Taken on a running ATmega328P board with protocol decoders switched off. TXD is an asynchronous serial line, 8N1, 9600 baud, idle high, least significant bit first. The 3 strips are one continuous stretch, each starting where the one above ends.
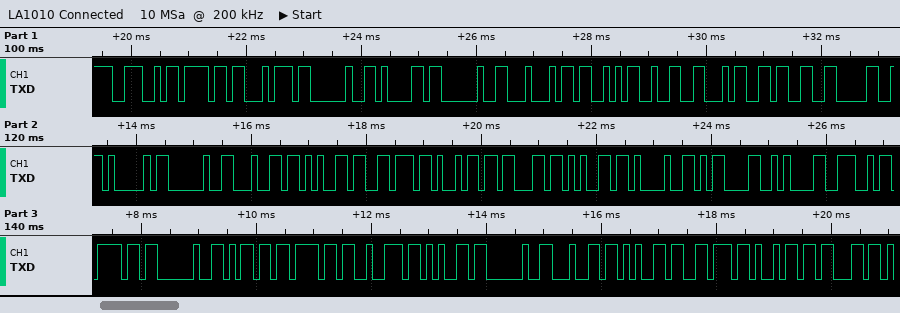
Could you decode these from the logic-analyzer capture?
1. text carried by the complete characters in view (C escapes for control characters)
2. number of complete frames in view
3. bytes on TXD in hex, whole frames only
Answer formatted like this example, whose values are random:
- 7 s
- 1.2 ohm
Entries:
- "Not a DS2430A device!\r\nNo more devic"
- 36
- 4E 6F 74 20 61 20 44 53 32 34 33 30 41 20 64 65 76 69 63 65 21 0D 0A 4E 6F 20 6D 6F 72 65 20 64 65 76 69 63
